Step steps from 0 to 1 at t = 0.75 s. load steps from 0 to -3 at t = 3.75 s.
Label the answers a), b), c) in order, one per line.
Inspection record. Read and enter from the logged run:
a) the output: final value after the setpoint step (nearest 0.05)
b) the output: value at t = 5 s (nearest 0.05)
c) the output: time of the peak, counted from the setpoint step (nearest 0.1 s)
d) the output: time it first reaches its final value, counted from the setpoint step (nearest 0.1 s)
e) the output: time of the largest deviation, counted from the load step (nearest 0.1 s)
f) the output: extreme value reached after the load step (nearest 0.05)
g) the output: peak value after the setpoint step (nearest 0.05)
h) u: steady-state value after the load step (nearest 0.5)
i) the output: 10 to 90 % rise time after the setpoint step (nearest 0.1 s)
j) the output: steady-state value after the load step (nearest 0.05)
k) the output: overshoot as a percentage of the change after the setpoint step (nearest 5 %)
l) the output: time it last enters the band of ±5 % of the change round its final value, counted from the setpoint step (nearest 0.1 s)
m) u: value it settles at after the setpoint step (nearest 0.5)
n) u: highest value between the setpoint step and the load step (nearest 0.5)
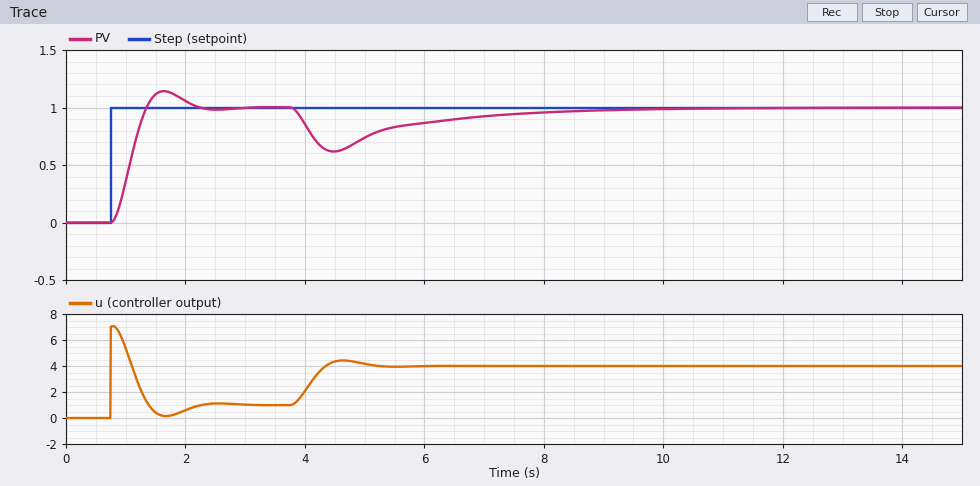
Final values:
a) 1.00
b) 0.75
c) 0.9 s
d) 0.6 s
e) 0.7 s
f) 0.60
g) 1.15
h) 4.0
i) 0.4 s
j) 1.00
k) 15 %
l) 1.3 s
m) 1.0
n) 7.0
